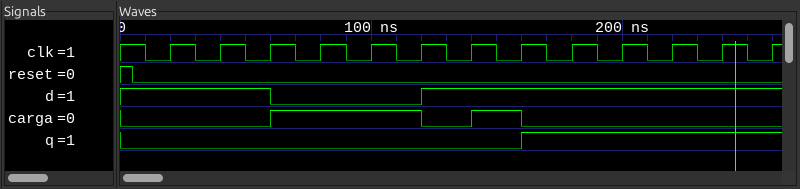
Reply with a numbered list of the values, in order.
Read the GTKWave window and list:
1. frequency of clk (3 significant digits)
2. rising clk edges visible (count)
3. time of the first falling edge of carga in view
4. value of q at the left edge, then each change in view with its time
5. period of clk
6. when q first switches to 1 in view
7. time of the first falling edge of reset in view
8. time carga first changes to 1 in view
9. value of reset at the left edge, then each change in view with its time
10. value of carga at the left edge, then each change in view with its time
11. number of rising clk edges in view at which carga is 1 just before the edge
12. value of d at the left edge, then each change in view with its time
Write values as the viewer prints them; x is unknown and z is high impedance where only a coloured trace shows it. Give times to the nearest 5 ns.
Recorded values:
1. 50.0 MHz
2. 13
3. 120 ns
4. 0, 1 at 160 ns
5. 20 ns
6. 160 ns
7. 5 ns
8. 60 ns
9. 1, 0 at 5 ns
10. 0, 1 at 60 ns, 0 at 120 ns, 1 at 140 ns, 0 at 160 ns
11. 4
12. 1, 0 at 60 ns, 1 at 120 ns
